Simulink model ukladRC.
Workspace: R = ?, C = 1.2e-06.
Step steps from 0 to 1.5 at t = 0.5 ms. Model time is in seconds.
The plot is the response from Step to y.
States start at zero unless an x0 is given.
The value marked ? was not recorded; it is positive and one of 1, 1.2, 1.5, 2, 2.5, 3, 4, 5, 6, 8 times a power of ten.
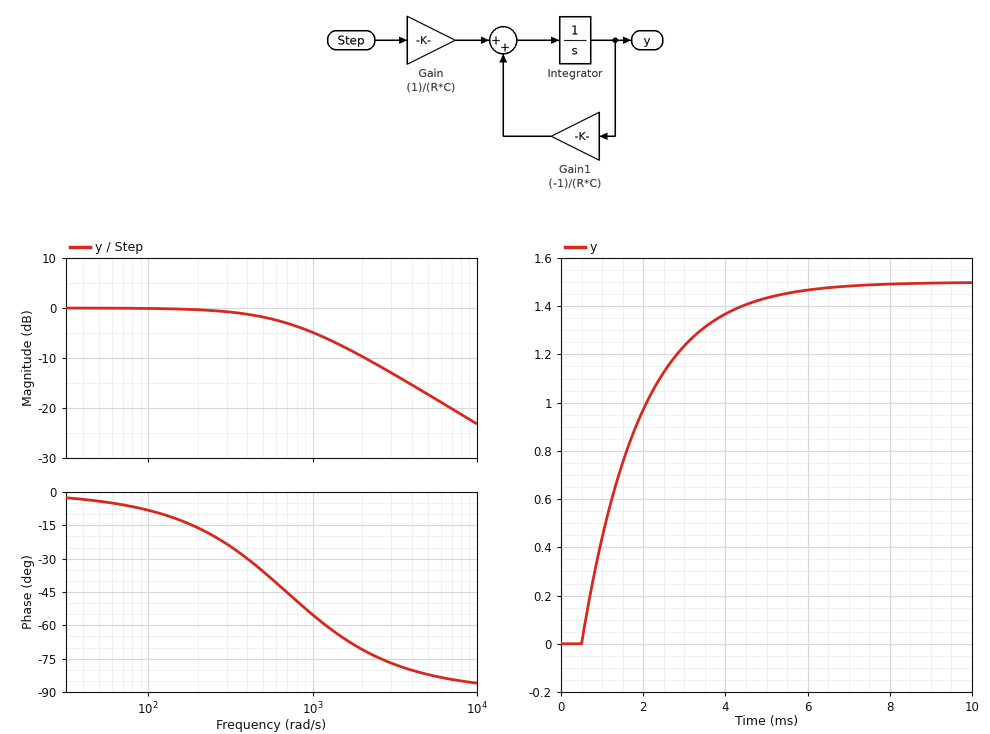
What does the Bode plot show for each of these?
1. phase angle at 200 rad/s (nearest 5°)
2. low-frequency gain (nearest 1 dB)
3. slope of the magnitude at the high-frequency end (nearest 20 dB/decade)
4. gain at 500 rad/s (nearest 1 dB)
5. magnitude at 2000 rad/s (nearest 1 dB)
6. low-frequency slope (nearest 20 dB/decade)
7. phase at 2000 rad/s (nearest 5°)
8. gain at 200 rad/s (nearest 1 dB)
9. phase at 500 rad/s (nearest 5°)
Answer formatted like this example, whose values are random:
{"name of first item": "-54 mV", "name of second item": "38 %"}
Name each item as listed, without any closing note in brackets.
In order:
{"phase angle at 200 rad/s": "-15°", "low-frequency gain": "0 dB", "slope of the magnitude at the high-frequency end": "-20 dB/decade", "gain at 500 rad/s": "-2 dB", "magnitude at 2000 rad/s": "-10 dB", "low-frequency slope": "0 dB/decade", "phase at 2000 rad/s": "-70°", "gain at 200 rad/s": "0 dB", "phase at 500 rad/s": "-35°"}
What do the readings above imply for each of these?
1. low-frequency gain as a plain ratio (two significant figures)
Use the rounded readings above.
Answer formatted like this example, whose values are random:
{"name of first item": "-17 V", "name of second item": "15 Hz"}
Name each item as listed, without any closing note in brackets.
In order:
{"low-frequency gain as a plain ratio": "1.0"}
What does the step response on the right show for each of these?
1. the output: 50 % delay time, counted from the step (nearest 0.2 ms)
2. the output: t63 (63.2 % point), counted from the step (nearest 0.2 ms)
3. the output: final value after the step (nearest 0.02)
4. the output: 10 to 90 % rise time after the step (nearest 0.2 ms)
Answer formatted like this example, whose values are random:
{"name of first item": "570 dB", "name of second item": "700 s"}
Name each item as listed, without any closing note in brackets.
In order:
{"the output: 50 % delay time, counted from the step": "1.0 ms", "the output: t63 (63.2 % point), counted from the step": "1.4 ms", "the output: final value after the step": "1.50", "the output: 10 to 90 % rise time after the step": "3.2 ms"}
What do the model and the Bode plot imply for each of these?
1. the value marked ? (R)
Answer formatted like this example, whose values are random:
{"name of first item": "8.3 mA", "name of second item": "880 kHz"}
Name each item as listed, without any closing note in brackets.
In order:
{"the value marked ?": "1200"}
